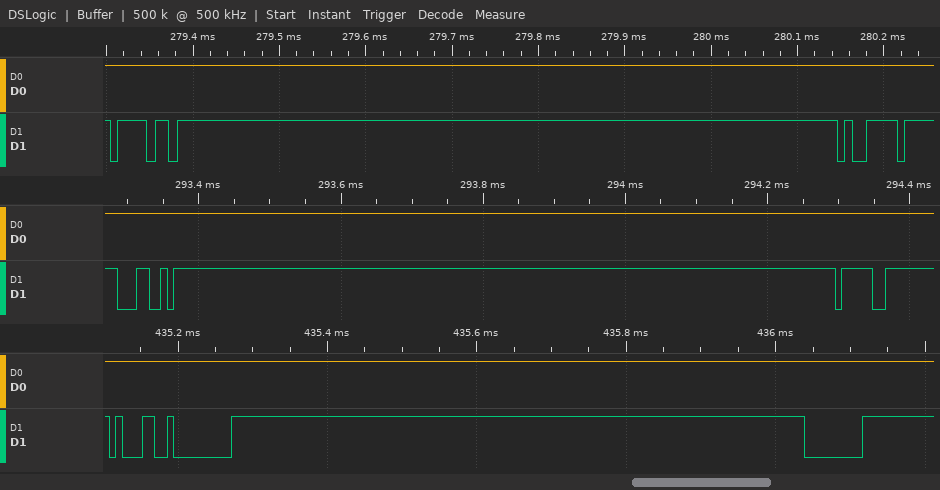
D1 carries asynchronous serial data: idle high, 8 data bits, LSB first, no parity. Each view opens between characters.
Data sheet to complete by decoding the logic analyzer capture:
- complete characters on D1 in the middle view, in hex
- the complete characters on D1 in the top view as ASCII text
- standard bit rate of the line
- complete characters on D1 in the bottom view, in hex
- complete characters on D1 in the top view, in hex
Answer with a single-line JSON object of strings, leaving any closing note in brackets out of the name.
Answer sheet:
{"complete characters on D1 in the middle view, in hex": "4C, 9F", "the complete characters on D1 in the top view as ASCII text": "\"oy\"", "standard bit rate of the line": "115200 baud", "complete characters on D1 in the bottom view, in hex": "31, 00, 00", "complete characters on D1 in the top view, in hex": "6F, 79"}
